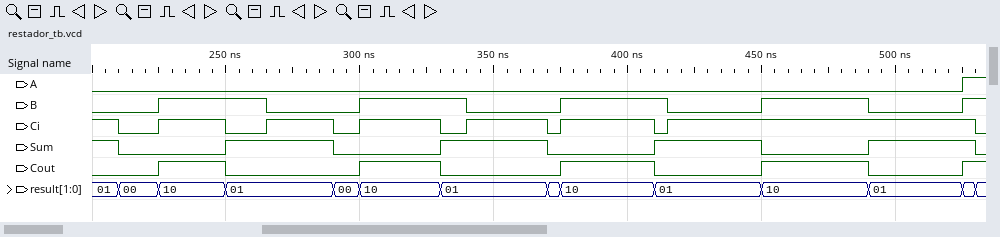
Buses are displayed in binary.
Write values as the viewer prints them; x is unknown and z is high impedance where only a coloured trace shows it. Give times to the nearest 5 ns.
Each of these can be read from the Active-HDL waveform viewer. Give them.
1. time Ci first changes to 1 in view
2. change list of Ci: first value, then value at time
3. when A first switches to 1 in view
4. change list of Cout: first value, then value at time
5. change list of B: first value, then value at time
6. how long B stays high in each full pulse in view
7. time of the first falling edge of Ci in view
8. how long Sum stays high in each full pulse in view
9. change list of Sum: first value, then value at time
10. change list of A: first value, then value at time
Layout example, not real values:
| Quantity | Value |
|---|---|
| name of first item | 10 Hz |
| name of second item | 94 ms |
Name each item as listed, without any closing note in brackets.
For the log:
| Quantity | Value |
|---|---|
| time Ci first changes to 1 in view | 225 ns |
| change list of Ci: first value, then value at time | 1, 0 at 210 ns, 1 at 225 ns, 0 at 250 ns, 1 at 265 ns, 0 at 290 ns, 1 at 300 ns, 0 at 330 ns, 1 at 340 ns, 0 at 370 ns, 1 at 375 ns, 0 at 410 ns, 1 at 415 ns, 0 at 530 ns |
| when A first switches to 1 in view | 525 ns |
| change list of Cout: first value, then value at time | 0, 1 at 225 ns, 0 at 250 ns, 1 at 300 ns, 0 at 330 ns, 1 at 375 ns, 0 at 410 ns, 1 at 450 ns, 0 at 490 ns, 1 at 525 ns |
| change list of B: first value, then value at time | 0, 1 at 225 ns, 0 at 265 ns, 1 at 300 ns, 0 at 340 ns, 1 at 375 ns, 0 at 415 ns, 1 at 450 ns, 0 at 490 ns, 1 at 525 ns |
| how long B stays high in each full pulse in view | 40 ns, 40 ns, 40 ns, 40 ns |
| time of the first falling edge of Ci in view | 210 ns |
| how long Sum stays high in each full pulse in view | 40 ns, 40 ns, 40 ns, 40 ns |
| change list of Sum: first value, then value at time | 1, 0 at 210 ns, 1 at 250 ns, 0 at 290 ns, 1 at 330 ns, 0 at 370 ns, 1 at 410 ns, 0 at 450 ns, 1 at 490 ns, 0 at 530 ns |
| change list of A: first value, then value at time | 0, 1 at 525 ns |
